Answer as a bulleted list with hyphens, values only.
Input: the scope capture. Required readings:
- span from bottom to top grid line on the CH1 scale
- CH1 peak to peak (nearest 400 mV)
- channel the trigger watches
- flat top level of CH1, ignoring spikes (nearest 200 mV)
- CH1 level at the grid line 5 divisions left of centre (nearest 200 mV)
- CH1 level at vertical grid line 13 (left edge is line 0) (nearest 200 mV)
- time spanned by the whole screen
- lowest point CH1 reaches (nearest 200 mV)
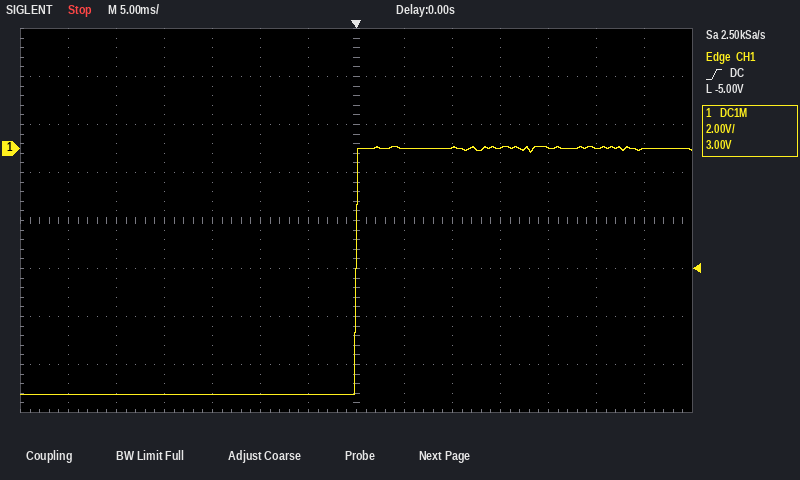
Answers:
- 16 V
- 10.4 V
- CH1
- 0.0 V
- -10.2 V
- 0.0 V
- 70 ms
- -10.2 V
